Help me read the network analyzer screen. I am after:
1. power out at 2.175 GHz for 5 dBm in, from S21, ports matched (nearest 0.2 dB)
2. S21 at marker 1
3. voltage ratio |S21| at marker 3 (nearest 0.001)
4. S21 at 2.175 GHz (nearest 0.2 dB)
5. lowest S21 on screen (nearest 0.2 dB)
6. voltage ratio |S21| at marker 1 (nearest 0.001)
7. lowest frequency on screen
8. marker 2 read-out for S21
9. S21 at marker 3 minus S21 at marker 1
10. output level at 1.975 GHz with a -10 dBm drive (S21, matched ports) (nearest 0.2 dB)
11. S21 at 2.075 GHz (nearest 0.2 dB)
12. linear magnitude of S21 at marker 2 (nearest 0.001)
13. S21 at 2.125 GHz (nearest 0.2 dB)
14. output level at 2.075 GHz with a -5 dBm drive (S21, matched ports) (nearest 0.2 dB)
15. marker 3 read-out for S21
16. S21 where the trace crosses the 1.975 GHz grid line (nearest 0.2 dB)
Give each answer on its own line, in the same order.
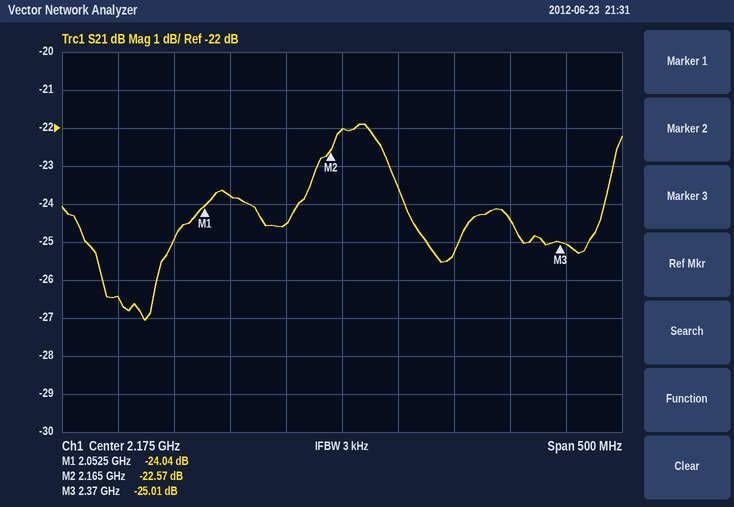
-17.0 dBm
-24.04 dB
0.056
-22.0 dB
-27.0 dB
0.063
1.925 GHz
-22.57 dB
-0.97 dB
-36.4 dBm
-23.8 dB
0.074
-24.6 dB
-28.8 dBm
-25.01 dB
-26.4 dB
